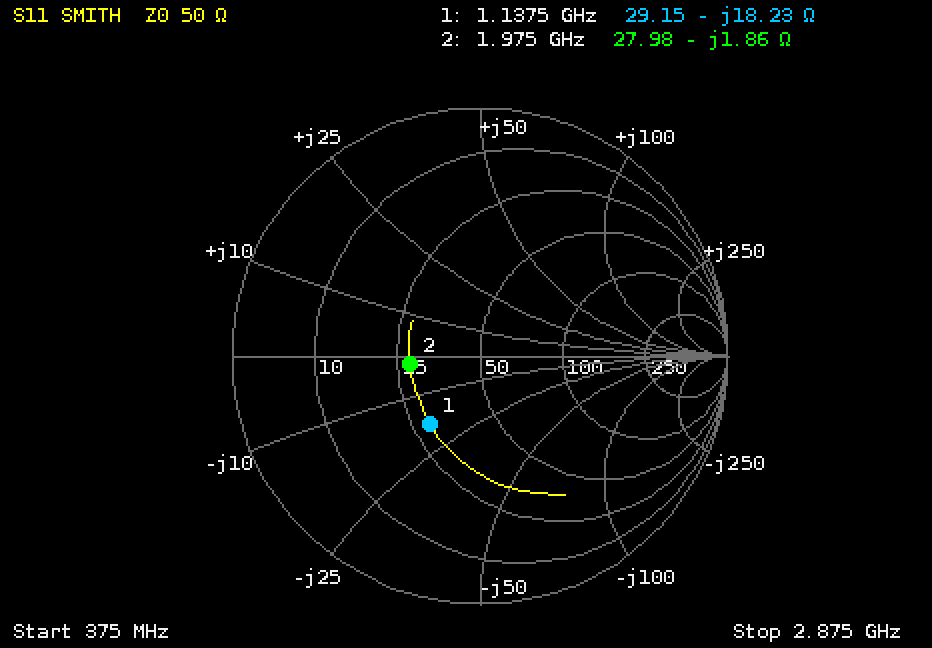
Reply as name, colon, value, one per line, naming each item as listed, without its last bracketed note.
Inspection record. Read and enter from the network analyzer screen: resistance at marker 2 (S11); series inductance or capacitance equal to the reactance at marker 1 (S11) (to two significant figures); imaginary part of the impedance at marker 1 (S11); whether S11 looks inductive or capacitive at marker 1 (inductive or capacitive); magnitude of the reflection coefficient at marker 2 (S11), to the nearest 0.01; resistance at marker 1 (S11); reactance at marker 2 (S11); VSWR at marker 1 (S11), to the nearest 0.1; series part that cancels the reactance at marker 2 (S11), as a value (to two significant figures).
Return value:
resistance at marker 2: 27.98 Ω
series inductance or capacitance equal to the reactance at marker 1 (S11): 7.7 pF
imaginary part of the impedance at marker 1: -18.23 Ω
whether S11 looks inductive or capacitive at marker 1: capacitive
magnitude of the reflection coefficient at marker 2 (S11), to the nearest 0.01: 0.28
resistance at marker 1: 29.15 Ω
reactance at marker 2: -1.86 Ω
VSWR at marker 1 (S11), to the nearest 0.1: 2.0
series part that cancels the reactance at marker 2 (S11), as a value: 150 pH
